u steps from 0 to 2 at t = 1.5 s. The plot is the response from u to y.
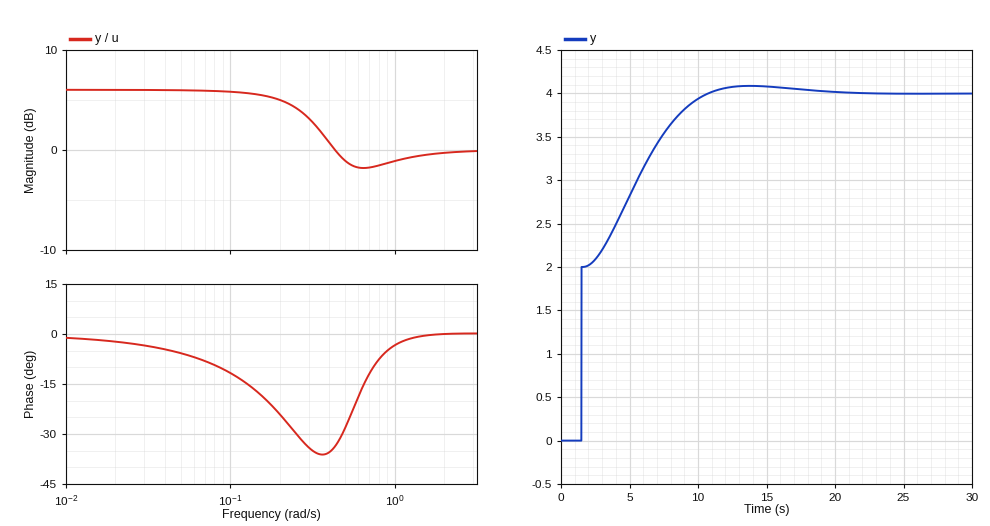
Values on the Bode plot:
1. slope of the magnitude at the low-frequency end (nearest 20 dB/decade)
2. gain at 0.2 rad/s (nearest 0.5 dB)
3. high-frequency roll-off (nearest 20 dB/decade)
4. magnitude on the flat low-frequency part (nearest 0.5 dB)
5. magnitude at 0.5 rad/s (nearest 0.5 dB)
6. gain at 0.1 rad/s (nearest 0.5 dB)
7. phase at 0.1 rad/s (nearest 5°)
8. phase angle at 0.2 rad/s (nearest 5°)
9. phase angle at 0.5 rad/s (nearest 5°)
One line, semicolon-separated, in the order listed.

0 dB/decade; 5.0 dB; 0 dB/decade; 6.0 dB; -1.0 dB; 6.0 dB; -10°; -25°; -30°
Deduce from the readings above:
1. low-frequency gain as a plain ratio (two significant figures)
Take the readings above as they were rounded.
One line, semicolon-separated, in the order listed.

2.0
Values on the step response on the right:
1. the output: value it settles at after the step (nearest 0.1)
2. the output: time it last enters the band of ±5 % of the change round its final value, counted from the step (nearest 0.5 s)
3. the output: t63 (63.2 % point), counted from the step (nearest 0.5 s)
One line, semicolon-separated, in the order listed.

4.0; 7.5 s; 2.5 s
